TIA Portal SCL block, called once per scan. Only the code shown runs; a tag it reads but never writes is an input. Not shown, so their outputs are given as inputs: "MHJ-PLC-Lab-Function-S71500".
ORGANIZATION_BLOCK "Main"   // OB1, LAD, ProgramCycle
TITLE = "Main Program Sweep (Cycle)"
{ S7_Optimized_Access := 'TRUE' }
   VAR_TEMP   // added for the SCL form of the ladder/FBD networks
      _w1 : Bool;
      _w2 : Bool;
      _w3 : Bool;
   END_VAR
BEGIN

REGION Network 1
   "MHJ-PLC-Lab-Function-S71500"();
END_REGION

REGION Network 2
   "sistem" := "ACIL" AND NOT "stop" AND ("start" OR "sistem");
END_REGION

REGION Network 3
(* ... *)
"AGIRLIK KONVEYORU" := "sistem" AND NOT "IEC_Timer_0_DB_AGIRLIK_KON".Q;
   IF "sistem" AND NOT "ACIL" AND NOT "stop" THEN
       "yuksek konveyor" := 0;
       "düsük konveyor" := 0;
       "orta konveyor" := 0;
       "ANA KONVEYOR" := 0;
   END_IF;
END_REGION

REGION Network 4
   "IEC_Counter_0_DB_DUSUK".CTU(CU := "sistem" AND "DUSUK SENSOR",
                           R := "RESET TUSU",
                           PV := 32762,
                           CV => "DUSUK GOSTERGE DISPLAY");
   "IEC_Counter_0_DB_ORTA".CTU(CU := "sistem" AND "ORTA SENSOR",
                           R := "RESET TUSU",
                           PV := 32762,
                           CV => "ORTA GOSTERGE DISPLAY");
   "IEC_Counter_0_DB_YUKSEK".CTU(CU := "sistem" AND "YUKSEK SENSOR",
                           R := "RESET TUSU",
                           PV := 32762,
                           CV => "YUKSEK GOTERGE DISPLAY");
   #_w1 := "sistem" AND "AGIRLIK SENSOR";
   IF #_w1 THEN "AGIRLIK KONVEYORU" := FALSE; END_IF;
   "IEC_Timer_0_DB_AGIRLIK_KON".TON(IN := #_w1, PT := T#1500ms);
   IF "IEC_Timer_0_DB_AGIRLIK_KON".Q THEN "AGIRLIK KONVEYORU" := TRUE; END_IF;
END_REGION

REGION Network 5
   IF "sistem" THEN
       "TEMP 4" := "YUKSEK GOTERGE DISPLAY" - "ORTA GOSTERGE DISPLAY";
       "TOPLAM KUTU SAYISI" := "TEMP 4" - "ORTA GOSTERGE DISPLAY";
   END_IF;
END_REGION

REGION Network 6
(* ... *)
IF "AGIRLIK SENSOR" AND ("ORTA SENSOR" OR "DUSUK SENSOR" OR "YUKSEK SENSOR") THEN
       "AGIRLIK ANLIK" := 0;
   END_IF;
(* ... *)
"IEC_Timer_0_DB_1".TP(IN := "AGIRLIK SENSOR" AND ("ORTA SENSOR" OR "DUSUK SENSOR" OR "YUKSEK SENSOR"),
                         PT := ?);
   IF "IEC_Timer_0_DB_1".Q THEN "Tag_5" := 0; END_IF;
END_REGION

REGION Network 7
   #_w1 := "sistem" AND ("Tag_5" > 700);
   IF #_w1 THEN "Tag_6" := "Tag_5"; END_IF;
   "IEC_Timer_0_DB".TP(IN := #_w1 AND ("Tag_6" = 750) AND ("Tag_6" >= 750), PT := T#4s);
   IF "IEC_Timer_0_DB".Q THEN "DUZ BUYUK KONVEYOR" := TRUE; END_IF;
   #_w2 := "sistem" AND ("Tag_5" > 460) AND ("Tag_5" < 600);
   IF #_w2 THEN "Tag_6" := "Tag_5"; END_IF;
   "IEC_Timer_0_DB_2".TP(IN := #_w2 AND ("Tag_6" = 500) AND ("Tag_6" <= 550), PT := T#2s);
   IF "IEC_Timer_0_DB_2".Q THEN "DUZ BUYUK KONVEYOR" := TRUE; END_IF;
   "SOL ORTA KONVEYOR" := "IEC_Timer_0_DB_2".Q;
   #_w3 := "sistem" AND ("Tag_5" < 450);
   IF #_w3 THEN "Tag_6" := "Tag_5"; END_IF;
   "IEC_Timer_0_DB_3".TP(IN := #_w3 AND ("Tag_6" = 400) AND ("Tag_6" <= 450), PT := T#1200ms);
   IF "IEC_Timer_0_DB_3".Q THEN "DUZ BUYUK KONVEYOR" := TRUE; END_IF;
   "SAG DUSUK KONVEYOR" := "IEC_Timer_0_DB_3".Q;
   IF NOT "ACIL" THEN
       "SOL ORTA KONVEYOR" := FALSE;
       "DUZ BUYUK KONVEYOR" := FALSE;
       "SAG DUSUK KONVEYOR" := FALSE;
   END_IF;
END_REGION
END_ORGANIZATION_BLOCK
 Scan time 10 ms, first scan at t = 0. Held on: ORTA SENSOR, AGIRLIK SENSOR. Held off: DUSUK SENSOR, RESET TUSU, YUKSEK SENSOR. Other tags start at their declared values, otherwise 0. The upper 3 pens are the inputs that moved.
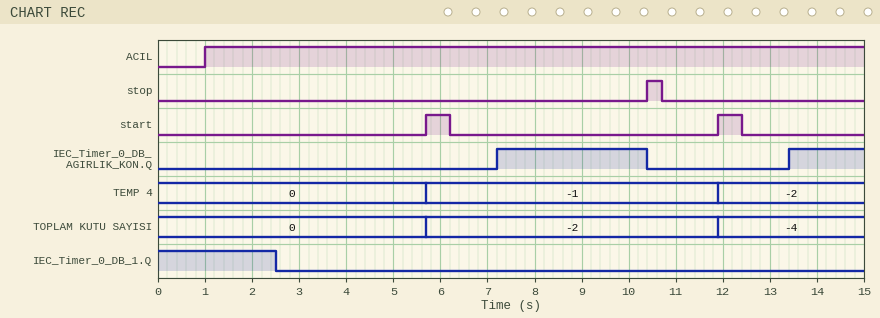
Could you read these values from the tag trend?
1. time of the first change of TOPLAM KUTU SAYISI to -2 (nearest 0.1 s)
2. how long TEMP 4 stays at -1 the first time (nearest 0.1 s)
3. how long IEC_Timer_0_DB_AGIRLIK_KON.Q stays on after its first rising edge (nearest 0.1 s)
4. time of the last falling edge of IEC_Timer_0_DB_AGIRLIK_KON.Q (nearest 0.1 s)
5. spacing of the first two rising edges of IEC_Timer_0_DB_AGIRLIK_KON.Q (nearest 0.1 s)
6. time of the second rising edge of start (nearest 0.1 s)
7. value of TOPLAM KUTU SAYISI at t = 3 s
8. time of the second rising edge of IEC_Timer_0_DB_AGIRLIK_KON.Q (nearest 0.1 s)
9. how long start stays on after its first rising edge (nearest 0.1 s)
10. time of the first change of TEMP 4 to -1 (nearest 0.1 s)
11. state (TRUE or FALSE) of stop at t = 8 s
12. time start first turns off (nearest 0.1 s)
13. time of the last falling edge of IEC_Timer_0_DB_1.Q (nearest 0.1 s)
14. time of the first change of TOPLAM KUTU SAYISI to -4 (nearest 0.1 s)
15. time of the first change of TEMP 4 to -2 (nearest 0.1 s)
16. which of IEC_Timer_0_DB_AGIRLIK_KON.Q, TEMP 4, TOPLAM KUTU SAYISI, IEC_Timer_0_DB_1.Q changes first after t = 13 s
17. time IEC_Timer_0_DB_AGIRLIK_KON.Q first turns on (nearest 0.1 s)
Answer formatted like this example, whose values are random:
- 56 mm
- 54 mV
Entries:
- 5.7 s
- 6.2 s
- 3.2 s
- 10.4 s
- 6.2 s
- 11.9 s
- 0
- 13.4 s
- 0.5 s
- 5.7 s
- FALSE
- 6.2 s
- 2.5 s
- 11.9 s
- 11.9 s
- IEC_Timer_0_DB_AGIRLIK_KON.Q
- 7.2 s
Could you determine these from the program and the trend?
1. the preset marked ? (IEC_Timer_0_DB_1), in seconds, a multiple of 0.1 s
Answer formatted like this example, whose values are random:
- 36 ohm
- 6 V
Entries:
- 2.5 s
